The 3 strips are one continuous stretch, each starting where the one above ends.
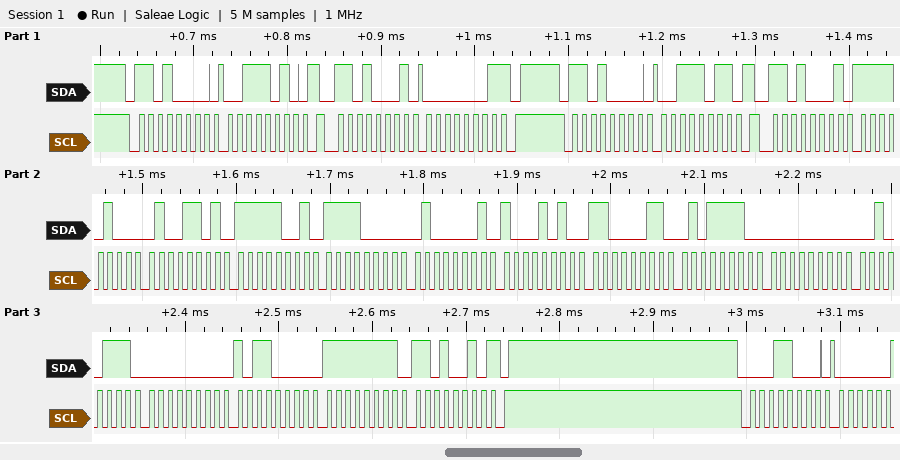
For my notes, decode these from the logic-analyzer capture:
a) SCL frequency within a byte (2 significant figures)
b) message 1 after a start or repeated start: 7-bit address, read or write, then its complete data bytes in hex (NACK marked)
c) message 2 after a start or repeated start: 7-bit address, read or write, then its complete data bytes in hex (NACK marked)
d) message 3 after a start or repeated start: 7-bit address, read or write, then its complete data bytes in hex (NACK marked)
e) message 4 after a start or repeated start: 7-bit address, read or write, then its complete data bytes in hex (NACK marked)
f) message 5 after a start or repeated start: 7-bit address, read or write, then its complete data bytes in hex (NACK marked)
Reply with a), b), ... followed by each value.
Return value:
a) 100 kHz
b) 0x68 write: 3A
c) 0x68 read: 01 NACK
d) 0x68 write: 3B
e) 0x68 read: F4 4D F9 F0 41 8A C3 5E 00 27 00 B0 FF D2 NACK
f) 0x0C write
